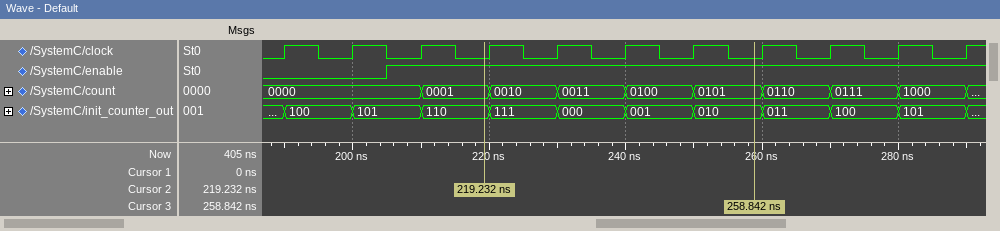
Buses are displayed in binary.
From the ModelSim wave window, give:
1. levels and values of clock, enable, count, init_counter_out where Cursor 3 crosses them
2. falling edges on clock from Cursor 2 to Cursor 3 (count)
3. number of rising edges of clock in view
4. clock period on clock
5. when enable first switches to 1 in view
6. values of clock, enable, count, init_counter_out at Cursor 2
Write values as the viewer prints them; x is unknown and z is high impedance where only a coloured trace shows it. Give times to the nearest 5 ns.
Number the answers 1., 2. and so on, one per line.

1. clock=0, enable=1, count=0101, init_counter_out=010
2. 4
3. 11
4. 10 ns
5. 205 ns
6. clock=0, enable=1, count=0001, init_counter_out=110
